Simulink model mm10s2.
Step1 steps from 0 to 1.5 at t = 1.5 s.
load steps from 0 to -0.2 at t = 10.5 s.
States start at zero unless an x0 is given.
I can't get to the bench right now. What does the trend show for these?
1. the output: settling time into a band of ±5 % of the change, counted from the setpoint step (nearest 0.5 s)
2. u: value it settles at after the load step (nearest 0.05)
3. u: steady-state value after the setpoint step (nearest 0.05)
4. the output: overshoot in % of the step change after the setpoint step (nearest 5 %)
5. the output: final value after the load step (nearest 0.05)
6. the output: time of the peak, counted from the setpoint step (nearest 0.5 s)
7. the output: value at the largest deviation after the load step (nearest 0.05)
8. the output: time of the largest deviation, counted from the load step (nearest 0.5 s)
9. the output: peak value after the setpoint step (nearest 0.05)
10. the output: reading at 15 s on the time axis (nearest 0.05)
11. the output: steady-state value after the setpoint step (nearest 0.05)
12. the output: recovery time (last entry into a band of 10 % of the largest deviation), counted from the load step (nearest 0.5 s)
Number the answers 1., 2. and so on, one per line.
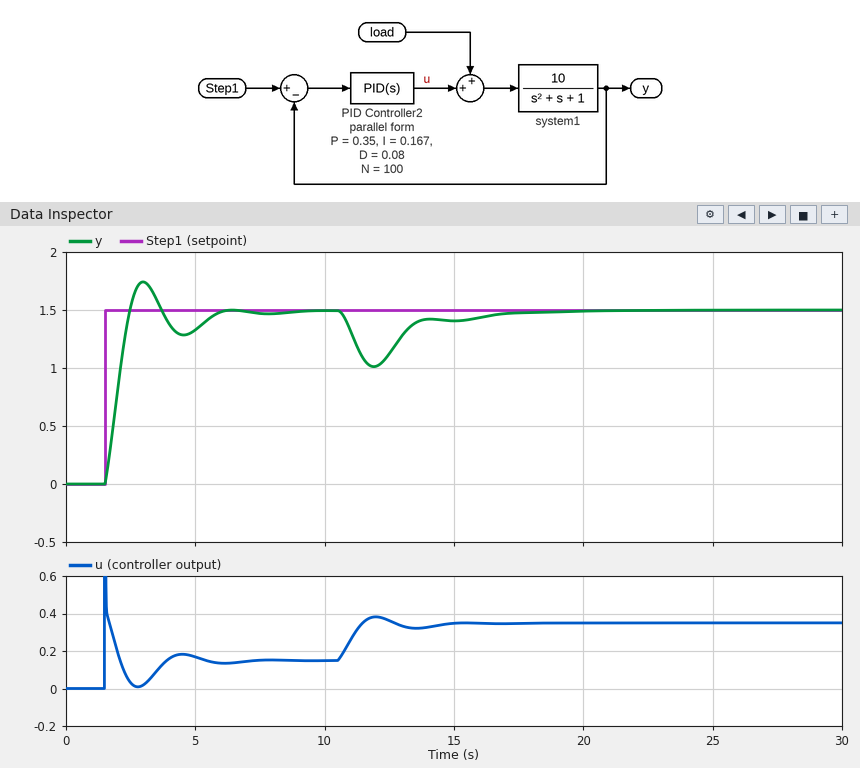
1. 4.0 s
2. 0.35
3. 0.15
4. 15 %
5. 1.50
6. 1.5 s
7. 1.00
8. 1.5 s
9. 1.75
10. 1.40
11. 1.50
12. 6.0 s
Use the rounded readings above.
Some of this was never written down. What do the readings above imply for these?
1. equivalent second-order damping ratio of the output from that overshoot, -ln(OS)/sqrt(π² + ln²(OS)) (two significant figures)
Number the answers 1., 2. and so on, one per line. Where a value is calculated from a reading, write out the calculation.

1. ln(0.15) = -1.897; 1.897 / sqrt(9.870 + 3.599) = 0.52
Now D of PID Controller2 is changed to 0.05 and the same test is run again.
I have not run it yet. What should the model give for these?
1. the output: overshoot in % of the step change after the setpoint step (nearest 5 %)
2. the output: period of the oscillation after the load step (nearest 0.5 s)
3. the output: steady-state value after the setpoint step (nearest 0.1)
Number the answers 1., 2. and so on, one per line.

1. 25 %
2. 3.0 s
3. 1.5
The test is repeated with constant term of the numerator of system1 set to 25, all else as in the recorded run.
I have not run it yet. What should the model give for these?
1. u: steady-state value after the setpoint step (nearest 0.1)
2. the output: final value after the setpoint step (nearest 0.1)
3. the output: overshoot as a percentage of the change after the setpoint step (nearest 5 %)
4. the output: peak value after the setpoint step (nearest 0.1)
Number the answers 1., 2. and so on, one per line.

1. 0.1
2. 1.5
3. 20 %
4. 1.8
